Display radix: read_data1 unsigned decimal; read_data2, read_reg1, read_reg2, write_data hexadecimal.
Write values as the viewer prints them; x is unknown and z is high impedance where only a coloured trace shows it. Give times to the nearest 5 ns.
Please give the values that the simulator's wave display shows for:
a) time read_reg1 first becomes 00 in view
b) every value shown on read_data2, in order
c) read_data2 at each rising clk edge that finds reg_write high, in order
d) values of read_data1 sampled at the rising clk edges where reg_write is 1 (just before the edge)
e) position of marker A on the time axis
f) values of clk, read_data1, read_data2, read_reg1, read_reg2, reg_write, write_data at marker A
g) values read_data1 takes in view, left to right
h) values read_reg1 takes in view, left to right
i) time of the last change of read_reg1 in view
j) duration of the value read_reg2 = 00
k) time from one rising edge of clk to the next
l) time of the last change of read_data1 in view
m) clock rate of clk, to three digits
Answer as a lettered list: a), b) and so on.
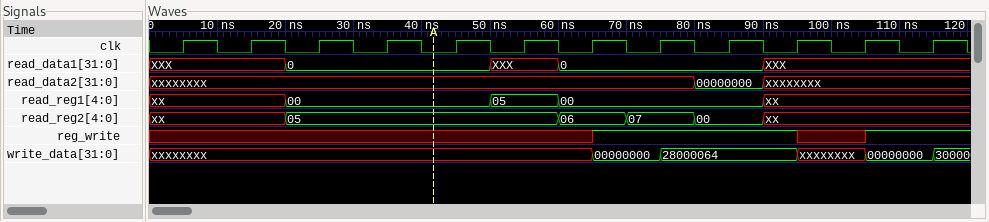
a) 20 ns
b) xxxxxxxx, 00000000, xxxxxxxx
c) xxxxxxxx, 00000000, xxxxxxxx, xxxxxxxx
d) 0, 0, XXX, XXX
e) 40 ns
f) clk=0, read_data1=0, read_data2=xxxxxxxx, read_reg1=00, read_reg2=05, reg_write=x, write_data=xxxxxxxx
g) XXX, 0, XXX, 0, XXX
h) xx, 00, 05, 00, xx
i) 90 ns
j) 10 ns
k) 10 ns
l) 90 ns
m) 100 MHz
